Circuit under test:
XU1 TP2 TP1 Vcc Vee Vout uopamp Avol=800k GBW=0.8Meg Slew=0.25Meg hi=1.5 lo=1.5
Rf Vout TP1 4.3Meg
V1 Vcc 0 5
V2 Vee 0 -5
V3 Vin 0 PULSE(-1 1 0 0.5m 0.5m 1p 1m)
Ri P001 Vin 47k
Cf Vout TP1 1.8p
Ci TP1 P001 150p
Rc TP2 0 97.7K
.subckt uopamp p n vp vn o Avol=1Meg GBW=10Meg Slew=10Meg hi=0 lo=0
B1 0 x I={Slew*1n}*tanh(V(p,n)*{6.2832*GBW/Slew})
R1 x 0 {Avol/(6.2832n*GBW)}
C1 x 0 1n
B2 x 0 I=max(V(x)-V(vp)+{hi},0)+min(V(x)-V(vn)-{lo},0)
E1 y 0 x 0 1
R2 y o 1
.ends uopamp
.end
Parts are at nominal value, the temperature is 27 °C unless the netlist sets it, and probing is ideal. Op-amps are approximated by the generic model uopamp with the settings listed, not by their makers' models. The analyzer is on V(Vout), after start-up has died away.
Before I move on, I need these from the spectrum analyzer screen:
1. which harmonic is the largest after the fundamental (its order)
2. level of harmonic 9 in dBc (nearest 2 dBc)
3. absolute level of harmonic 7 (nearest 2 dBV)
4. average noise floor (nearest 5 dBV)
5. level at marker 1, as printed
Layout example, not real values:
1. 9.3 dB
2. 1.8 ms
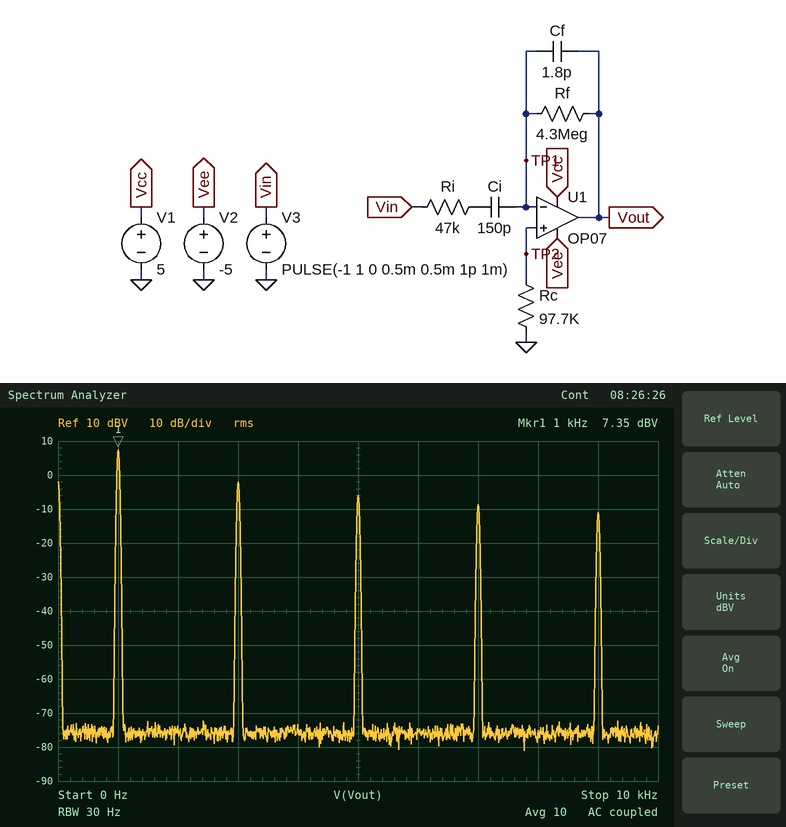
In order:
1. 3
2. -18 dBc
3. -8 dBV
4. -75 dBV
5. 7.35 dBV
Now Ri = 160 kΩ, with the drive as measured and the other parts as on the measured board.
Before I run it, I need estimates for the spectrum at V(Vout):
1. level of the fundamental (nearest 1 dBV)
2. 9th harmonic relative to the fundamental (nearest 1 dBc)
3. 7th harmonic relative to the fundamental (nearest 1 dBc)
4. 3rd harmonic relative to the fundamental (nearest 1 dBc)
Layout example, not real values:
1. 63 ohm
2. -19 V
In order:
1. 7 dBV
2. -24 dBc
3. -20 dBc
4. -10 dBc
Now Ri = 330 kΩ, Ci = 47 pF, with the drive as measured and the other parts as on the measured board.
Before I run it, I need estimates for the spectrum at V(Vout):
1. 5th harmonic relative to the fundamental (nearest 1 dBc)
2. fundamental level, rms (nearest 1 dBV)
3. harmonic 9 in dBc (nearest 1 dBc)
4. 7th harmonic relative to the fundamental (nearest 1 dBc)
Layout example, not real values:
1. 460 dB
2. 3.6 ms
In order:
1. -15 dBc
2. -3 dBV
3. -22 dBc
4. -19 dBc
